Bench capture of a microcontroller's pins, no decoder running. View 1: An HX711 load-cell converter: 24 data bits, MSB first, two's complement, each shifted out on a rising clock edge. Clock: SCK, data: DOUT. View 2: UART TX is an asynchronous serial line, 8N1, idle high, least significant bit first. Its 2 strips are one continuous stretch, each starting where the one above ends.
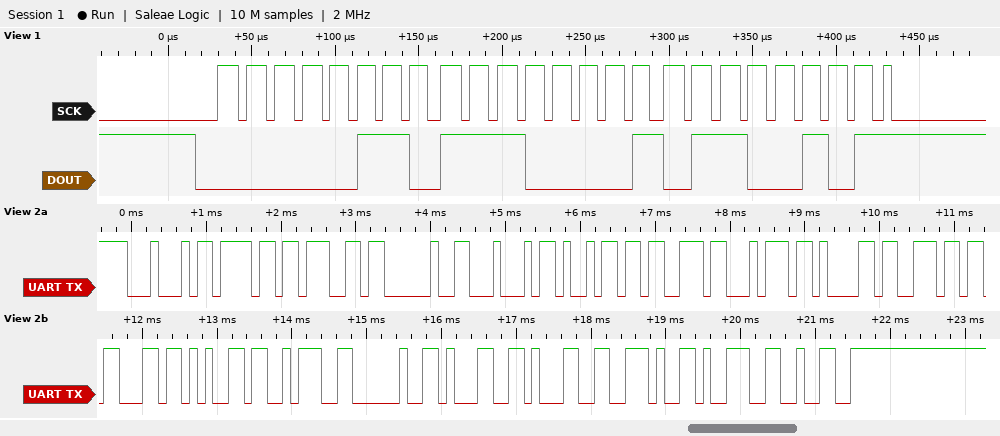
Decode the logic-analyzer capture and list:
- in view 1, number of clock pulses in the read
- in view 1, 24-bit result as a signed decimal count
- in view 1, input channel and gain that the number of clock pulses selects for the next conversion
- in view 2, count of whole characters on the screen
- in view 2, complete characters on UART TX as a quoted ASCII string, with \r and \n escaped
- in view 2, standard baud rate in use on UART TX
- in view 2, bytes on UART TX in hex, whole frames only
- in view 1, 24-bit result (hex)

25
450917
channel A, gain 128
19
"Dog Distance: 11.92"
9600 baud
0x44 0x6F 0x67 0x20 0x44 0x69 0x73 0x74 0x61 0x6E 0x63 0x65 0x3A 0x20 0x31 0x31 0x2E 0x39 0x32
0x06E165
